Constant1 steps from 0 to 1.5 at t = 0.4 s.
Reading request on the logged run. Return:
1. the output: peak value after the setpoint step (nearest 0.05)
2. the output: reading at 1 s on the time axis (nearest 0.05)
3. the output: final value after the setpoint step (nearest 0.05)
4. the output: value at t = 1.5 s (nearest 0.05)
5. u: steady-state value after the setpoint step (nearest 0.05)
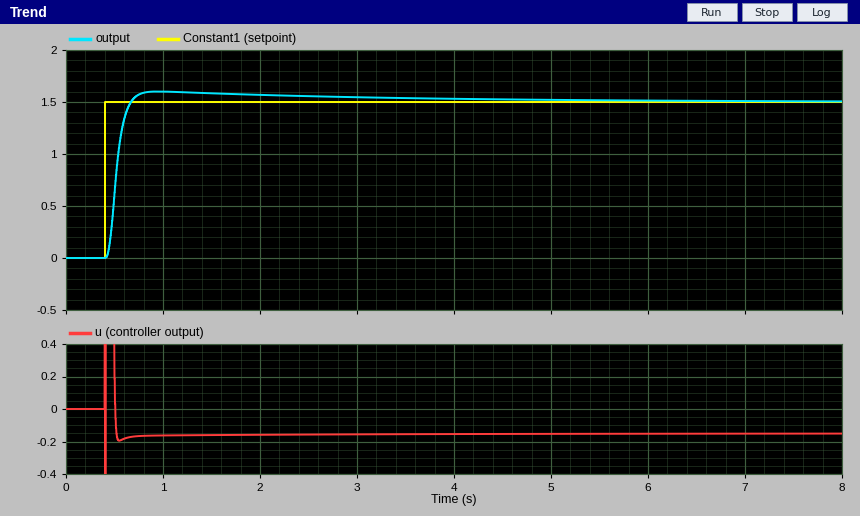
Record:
1.60
1.60
1.50
1.60
-0.15
